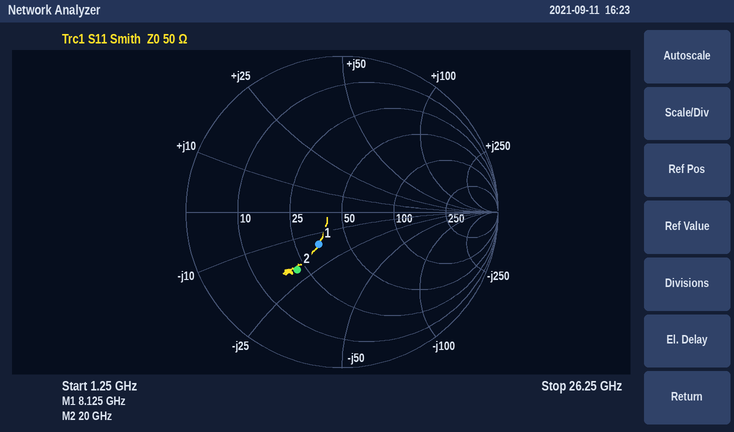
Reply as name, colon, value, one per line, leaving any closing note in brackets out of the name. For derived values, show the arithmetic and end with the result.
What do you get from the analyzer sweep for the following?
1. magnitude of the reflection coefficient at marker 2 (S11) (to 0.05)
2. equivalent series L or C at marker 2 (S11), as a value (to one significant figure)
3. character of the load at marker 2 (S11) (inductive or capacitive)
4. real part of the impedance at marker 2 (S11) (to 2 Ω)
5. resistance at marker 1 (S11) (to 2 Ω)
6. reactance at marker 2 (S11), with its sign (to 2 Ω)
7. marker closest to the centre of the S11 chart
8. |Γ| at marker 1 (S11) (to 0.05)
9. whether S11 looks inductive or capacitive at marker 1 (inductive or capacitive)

magnitude of the reflection coefficient at marker 2 (S11): 0.45
equivalent series L or C at marker 2 (S11), as a value: C = 1/(2π × 20 GHz × 20 Ω) ≈ 398 fF, so 400 fF to one significant figure
character of the load at marker 2 (S11): capacitive
real part of the impedance at marker 2 (S11): 22 Ω
resistance at marker 1 (S11): 34 Ω
reactance at marker 2 (S11), with its sign: -20 Ω
marker closest to the centre of the S11 chart: marker 1
|Γ| at marker 1 (S11): 0.25
whether S11 looks inductive or capacitive at marker 1: capacitive
